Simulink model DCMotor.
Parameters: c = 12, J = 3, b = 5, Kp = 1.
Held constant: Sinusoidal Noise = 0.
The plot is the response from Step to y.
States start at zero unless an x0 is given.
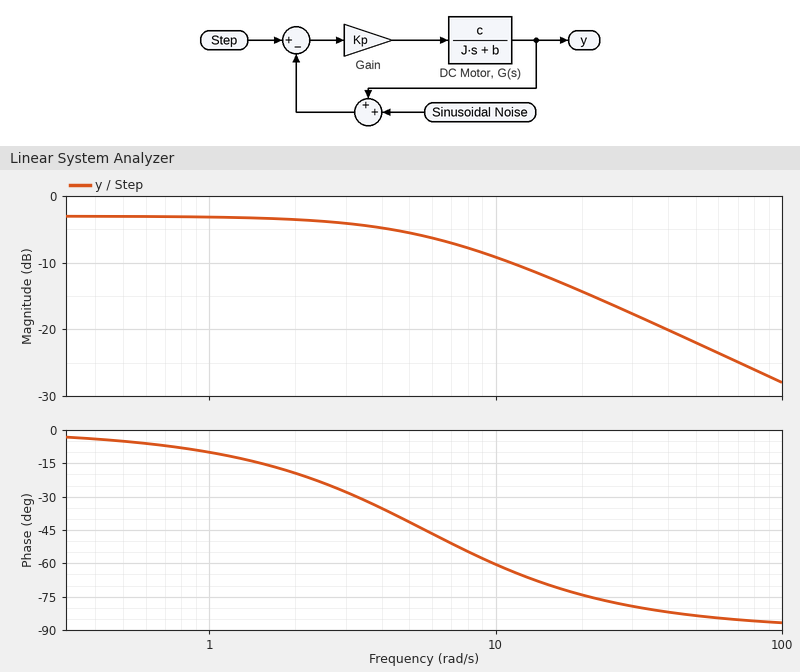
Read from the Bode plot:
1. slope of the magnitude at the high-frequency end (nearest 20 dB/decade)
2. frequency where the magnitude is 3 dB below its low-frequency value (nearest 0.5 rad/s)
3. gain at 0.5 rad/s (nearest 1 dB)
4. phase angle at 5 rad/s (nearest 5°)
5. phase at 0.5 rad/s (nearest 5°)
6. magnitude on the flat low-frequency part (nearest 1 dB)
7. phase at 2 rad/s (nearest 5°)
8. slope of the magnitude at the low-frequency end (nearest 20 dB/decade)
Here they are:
-20 dB/decade
5.5 rad/s
-3 dB
-40°
-5°
-3 dB
-20°
0 dB/decade
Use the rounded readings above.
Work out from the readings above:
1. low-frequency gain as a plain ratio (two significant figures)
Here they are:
0.71
